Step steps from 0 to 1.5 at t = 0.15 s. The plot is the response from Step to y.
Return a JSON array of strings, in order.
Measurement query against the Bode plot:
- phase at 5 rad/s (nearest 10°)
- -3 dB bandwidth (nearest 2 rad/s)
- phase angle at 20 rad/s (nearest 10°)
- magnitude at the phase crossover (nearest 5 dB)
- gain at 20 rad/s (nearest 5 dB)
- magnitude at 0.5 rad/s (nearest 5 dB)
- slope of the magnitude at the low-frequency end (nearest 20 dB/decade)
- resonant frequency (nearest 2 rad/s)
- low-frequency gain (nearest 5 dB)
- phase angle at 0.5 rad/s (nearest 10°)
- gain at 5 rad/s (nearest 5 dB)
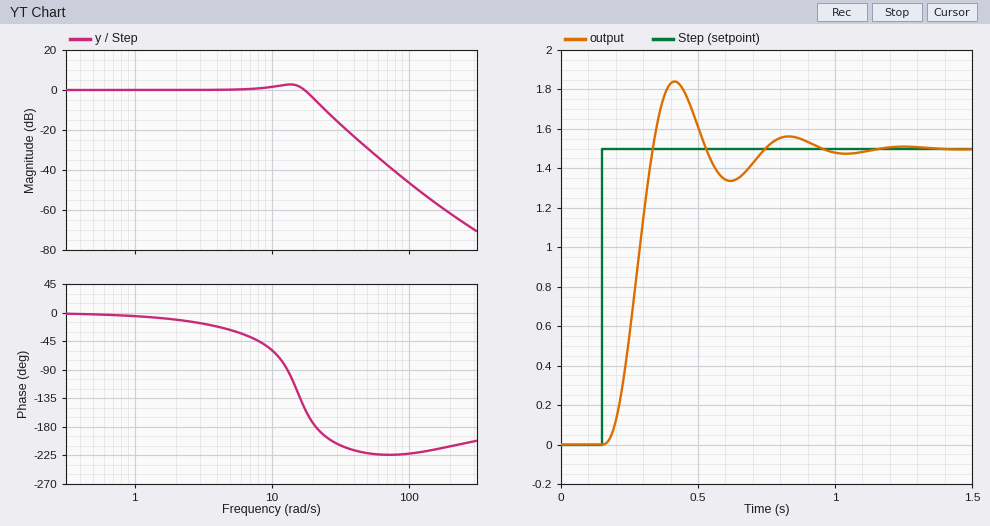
["-30°", "20 rad/s", "-170°", "-5 dB", "-5 dB", "0 dB", "0 dB/decade", "14 rad/s", "0 dB", "0°", "0 dB"]
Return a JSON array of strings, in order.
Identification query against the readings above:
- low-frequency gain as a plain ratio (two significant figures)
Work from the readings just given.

["1.0"]
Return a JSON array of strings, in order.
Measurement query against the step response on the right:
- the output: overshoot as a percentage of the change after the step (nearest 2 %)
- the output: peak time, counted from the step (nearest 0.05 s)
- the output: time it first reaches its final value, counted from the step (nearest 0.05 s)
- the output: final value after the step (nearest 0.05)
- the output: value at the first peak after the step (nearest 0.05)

["22 %", "0.25 s", "0.20 s", "1.50", "1.85"]
